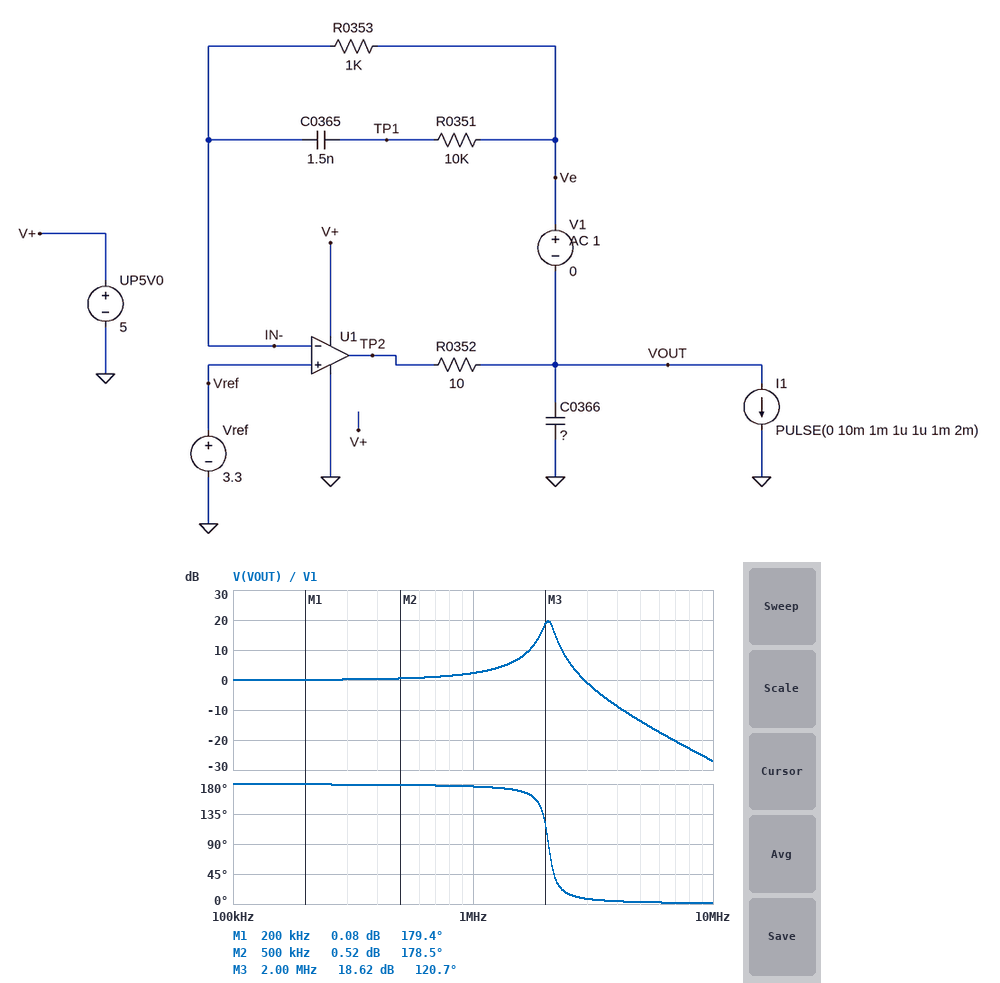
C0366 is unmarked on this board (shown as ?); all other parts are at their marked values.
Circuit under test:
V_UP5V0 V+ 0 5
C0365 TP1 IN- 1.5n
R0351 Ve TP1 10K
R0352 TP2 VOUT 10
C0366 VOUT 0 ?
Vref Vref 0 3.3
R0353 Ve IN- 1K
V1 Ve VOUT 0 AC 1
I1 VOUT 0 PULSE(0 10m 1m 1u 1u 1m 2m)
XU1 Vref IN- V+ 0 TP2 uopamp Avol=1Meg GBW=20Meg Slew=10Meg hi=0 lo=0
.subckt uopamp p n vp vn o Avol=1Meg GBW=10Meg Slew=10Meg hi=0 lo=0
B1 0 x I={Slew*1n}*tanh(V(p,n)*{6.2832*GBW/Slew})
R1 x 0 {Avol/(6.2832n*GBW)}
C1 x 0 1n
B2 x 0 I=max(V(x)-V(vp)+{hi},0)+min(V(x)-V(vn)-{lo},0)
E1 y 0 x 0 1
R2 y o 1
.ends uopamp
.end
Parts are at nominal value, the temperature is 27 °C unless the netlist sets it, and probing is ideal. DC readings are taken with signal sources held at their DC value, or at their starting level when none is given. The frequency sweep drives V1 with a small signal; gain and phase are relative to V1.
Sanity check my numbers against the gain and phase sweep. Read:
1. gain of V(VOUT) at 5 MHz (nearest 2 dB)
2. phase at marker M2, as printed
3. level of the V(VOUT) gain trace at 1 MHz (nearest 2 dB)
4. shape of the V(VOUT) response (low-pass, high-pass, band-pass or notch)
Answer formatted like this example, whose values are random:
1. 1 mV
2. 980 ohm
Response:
1. -14 dB
2. 178.5 deg
3. 2 dB
4. low-pass
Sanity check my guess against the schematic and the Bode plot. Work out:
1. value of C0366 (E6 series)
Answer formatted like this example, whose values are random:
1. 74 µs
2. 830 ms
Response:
1. 68 nF
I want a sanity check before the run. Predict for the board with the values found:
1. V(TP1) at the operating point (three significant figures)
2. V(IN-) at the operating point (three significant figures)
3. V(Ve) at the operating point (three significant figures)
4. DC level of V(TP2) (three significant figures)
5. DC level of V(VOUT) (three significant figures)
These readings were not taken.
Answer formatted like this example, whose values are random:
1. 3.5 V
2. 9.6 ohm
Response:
1. 3.30 V
2. 3.30 V
3. 3.30 V
4. 3.30 V
5. 3.30 V
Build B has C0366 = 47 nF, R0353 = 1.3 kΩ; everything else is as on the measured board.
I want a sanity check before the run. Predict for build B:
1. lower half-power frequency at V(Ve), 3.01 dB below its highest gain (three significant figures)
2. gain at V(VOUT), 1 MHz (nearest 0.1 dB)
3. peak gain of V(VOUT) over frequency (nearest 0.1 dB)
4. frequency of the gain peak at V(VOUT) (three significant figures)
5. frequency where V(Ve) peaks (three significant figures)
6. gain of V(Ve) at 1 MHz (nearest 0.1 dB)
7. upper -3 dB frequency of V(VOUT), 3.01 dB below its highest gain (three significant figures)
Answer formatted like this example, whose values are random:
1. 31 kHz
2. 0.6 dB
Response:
1. 2.35 MHz
2. 1.5 dB
3. 18.1 dB
4. 2.47 MHz
5. 2.49 MHz
6. -13.9 dB
7. 2.62 MHz
